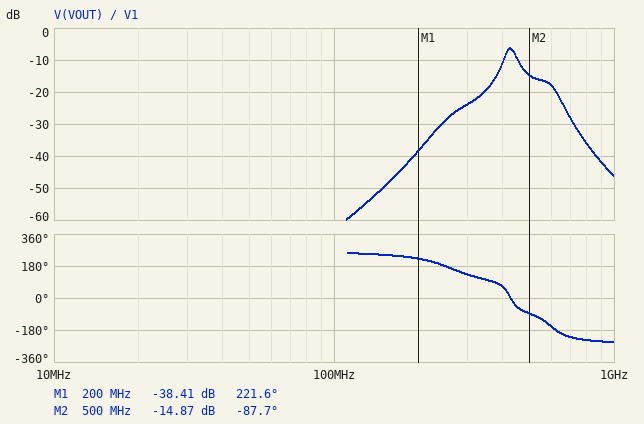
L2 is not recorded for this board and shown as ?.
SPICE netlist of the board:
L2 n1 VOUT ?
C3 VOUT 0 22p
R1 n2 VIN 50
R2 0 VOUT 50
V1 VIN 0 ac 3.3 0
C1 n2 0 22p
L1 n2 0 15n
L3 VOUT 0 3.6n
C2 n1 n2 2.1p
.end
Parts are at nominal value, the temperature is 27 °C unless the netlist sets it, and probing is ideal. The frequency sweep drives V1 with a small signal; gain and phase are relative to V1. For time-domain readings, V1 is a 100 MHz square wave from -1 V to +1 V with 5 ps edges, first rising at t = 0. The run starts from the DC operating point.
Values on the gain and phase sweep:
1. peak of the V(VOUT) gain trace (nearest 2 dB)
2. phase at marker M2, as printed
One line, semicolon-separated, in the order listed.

-6 dB; -87.7 deg
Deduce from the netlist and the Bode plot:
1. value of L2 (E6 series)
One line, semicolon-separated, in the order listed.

68 nH
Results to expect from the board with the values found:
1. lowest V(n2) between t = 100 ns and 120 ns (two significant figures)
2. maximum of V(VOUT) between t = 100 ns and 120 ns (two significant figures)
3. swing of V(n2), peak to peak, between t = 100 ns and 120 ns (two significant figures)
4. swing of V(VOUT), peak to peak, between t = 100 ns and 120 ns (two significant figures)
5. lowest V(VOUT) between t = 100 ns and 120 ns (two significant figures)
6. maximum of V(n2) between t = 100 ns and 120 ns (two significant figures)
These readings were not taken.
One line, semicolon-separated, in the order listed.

-660 mV; 75 mV; 1.3 V; 150 mV; -75 mV; 660 mV
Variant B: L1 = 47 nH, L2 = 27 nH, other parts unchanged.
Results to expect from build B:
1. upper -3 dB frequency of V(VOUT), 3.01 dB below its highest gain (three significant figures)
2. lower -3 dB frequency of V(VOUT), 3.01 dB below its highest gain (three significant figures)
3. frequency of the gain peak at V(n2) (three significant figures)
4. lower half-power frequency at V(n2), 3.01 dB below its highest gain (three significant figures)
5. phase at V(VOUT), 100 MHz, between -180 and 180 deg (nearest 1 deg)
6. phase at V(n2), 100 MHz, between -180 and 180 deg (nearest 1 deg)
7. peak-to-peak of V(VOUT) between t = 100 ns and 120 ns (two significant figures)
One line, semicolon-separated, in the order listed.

780 MHz; 727 MHz; 149 MHz; 97.4 MHz; -140 deg; 43 deg; 190 mV
